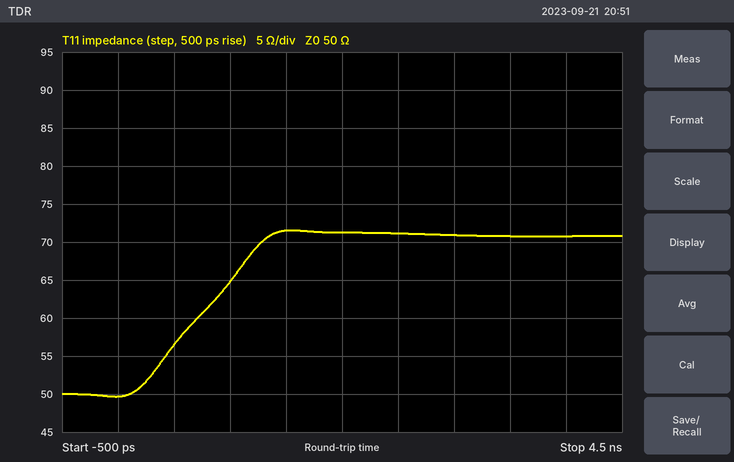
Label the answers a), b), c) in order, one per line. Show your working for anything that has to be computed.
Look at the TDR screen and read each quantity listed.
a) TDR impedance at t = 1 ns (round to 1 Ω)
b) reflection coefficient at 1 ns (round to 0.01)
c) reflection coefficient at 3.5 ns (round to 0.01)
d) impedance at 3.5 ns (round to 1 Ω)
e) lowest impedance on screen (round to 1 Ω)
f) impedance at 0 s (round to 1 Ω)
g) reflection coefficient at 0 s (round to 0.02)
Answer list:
a) 65 Ω
b) (65 − 50)/(65 + 50) ≈ +0.13
c) (71 − 50)/(71 + 50) ≈ +0.17
d) 71 Ω
e) 50 Ω
f) 50 Ω
g) (50 − 50)/(50 + 50) ≈ 0.00
